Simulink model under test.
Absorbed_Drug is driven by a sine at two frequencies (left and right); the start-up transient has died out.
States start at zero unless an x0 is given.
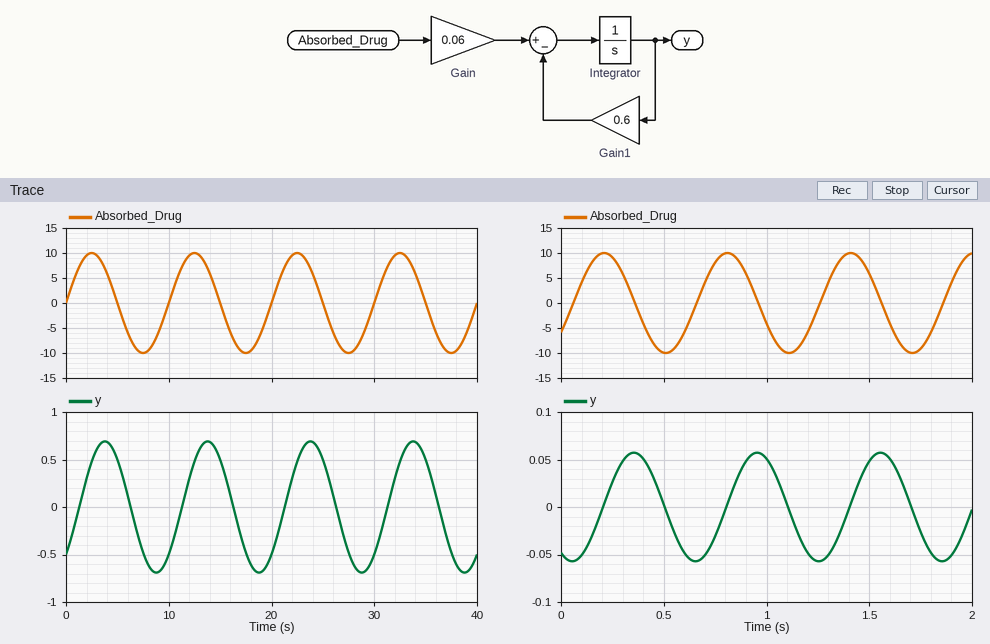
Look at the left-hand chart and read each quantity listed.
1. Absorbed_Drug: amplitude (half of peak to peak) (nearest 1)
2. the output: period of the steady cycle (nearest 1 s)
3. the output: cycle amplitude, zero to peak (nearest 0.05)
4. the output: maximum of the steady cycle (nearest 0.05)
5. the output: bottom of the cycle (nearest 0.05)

10
10 s
0.70
0.70
-0.70
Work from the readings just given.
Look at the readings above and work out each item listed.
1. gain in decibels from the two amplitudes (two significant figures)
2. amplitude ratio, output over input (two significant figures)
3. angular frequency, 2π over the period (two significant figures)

-23 dB
0.070
0.63 rad/s
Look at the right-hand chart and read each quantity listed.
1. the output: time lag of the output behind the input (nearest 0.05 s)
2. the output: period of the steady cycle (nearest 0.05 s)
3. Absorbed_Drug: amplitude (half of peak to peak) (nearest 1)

0.15 s
0.60 s
10
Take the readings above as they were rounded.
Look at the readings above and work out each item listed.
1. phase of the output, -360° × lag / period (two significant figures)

-90°
